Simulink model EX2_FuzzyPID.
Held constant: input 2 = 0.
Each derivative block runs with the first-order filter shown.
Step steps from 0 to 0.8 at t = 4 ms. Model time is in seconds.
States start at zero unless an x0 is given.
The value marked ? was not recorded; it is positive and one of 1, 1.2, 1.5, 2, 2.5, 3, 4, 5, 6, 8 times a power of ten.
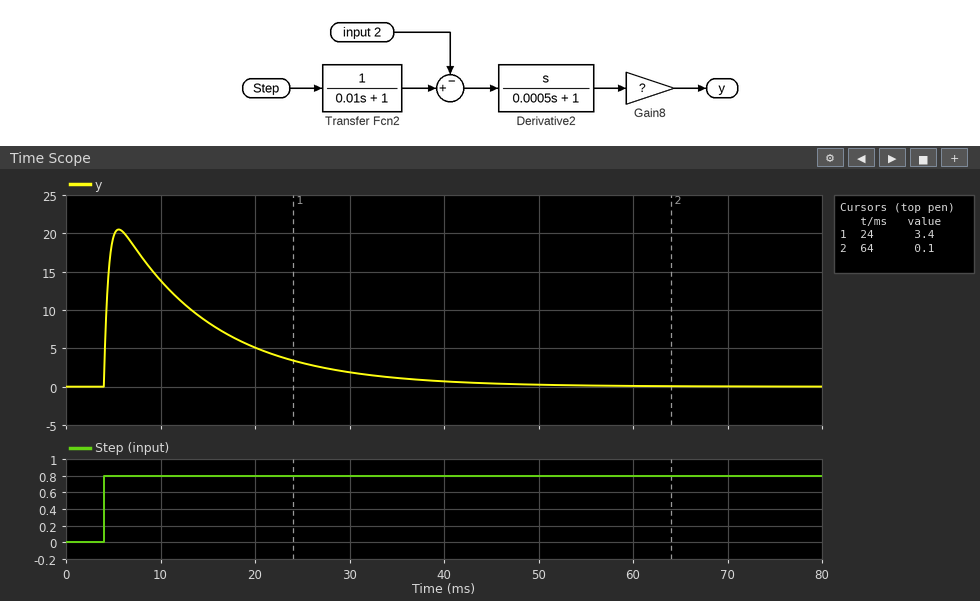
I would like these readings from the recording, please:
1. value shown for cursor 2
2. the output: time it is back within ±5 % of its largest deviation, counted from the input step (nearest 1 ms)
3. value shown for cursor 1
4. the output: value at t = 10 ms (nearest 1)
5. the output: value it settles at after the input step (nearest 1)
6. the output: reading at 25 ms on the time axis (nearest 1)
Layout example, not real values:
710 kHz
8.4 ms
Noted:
0.1
32 ms
3.4
14
0
3
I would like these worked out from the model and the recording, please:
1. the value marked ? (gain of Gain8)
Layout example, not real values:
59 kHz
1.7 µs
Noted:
0.3
